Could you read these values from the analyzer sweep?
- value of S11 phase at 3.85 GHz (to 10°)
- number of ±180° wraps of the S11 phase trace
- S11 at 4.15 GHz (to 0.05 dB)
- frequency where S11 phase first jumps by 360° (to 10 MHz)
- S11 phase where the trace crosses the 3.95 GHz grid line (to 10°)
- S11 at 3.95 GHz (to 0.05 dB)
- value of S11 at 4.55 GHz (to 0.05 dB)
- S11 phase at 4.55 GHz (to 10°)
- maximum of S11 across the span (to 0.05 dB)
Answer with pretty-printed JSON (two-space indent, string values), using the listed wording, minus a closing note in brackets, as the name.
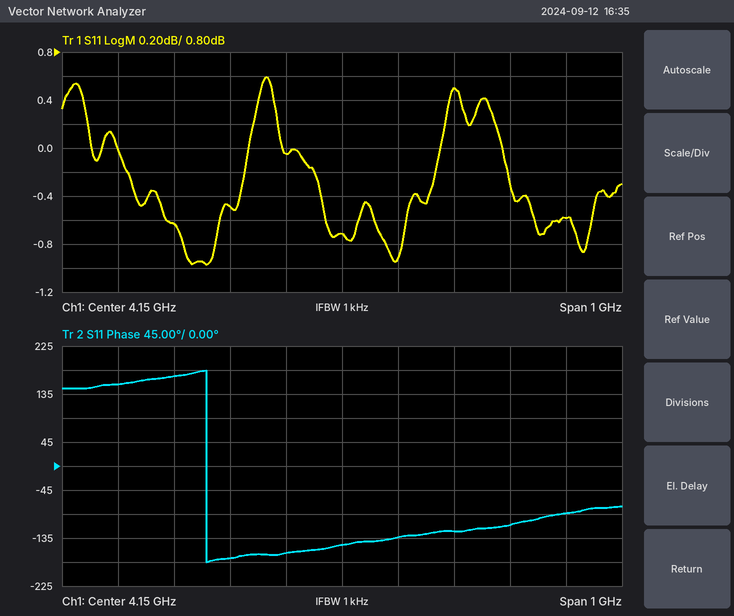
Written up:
{
  "value of S11 phase at 3.85 GHz": "170°",
  "number of ±180° wraps of the S11 phase trace": "1",
  "S11 at 4.15 GHz": "-0.70 dB",
  "frequency where S11 phase first jumps by 360°": "3.91 GHz",
  "S11 phase where the trace crosses the 3.95 GHz grid line": "-170°",
  "S11 at 3.95 GHz": "-0.50 dB",
  "value of S11 at 4.55 GHz": "-0.60 dB",
  "S11 phase at 4.55 GHz": "-90°",
  "maximum of S11 across the span": "0.60 dB"
}
